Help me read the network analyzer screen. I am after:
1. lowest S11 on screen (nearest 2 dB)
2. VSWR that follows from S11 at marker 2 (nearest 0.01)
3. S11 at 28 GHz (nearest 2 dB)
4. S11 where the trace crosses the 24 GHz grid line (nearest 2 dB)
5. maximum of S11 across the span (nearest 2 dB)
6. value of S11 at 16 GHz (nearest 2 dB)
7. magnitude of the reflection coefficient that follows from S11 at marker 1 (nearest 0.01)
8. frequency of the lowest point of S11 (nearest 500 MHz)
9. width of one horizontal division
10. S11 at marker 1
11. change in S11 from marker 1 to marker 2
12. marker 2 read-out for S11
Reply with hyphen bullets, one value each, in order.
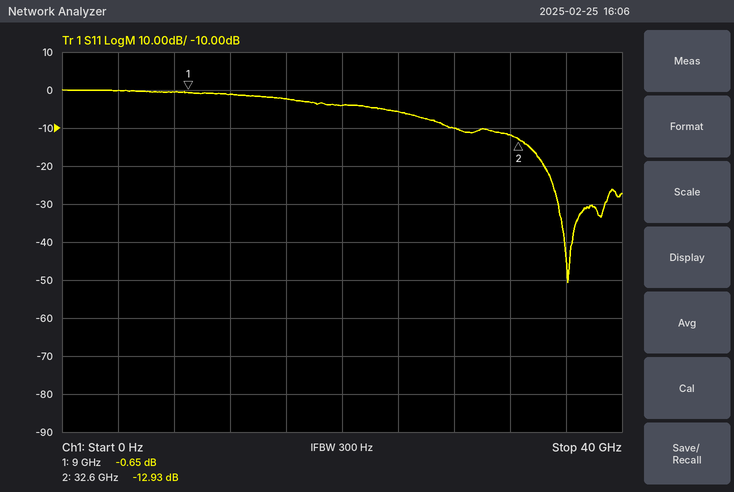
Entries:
- -50 dB
- 1.58
- -10 dB
- -6 dB
- 0 dB
- -2 dB
- 0.93
- 36.0 GHz
- 4 GHz
- -0.65 dB
- -12.28 dB
- -12.93 dB
